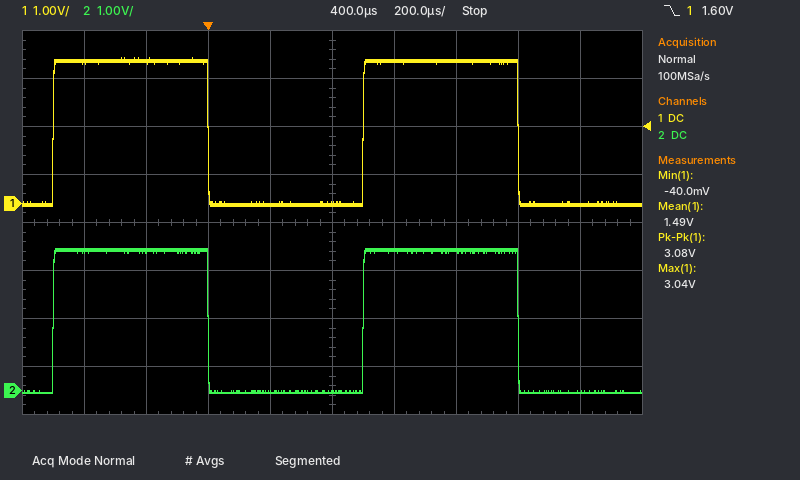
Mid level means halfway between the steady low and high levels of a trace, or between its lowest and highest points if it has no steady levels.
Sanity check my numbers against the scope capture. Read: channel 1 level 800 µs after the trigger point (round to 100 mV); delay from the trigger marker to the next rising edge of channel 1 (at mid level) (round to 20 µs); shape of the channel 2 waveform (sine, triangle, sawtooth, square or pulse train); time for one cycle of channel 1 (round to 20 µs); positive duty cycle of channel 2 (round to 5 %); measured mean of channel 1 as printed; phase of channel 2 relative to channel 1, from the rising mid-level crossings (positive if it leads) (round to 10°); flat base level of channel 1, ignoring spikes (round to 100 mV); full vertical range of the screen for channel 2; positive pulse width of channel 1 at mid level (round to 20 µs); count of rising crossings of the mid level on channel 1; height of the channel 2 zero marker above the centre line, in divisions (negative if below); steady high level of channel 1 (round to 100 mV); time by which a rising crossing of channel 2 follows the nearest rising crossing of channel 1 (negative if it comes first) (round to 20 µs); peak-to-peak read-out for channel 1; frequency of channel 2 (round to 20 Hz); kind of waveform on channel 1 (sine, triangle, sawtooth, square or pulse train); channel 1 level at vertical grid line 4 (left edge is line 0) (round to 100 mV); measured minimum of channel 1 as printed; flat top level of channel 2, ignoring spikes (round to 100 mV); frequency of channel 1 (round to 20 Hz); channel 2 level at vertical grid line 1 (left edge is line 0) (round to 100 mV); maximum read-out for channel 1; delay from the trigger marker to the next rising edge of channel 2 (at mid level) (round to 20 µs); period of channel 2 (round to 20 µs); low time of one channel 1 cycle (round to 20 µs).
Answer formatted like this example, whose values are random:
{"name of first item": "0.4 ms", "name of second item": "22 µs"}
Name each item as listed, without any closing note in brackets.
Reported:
{"channel 1 level 800 µs after the trigger point": "3.0 V", "delay from the trigger marker to the next rising edge of channel 1 (at mid level)": "500 µs", "shape of the channel 2 waveform": "square", "time for one cycle of channel 1": "1.00 ms", "positive duty cycle of channel 2": "50 %", "measured mean of channel 1 as printed": "1.49 V", "phase of channel 2 relative to channel 1, from the rising mid-level crossings (positive if it leads)": "0°", "flat base level of channel 1, ignoring spikes": "0.0 V", "full vertical range of the screen for channel 2": "8 V", "positive pulse width of channel 1 at mid level": "500 µs", "count of rising crossings of the mid level on channel 1": "2", "height of the channel 2 zero marker above the centre line, in divisions": "-3.5 div", "steady high level of channel 1": "3.0 V", "time by which a rising crossing of channel 2 follows the nearest rising crossing of channel 1 (negative if it comes first)": "0 µs", "peak-to-peak read-out for channel 1": "3.08 V", "frequency of channel 2": "1.00 kHz", "kind of waveform on channel 1": "square", "channel 1 level at vertical grid line 4 (left edge is line 0)": "0.0 V", "measured minimum of channel 1 as printed": "-40.0 mV", "flat top level of channel 2, ignoring spikes": "2.9 V", "frequency of channel 1": "1.00 kHz", "channel 2 level at vertical grid line 1 (left edge is line 0)": "2.9 V", "maximum read-out for channel 1": "3.04 V", "delay from the trigger marker to the next rising edge of channel 2 (at mid level)": "500 µs", "period of channel 2": "1.00 ms", "low time of one channel 1 cycle": "500 µs"}
